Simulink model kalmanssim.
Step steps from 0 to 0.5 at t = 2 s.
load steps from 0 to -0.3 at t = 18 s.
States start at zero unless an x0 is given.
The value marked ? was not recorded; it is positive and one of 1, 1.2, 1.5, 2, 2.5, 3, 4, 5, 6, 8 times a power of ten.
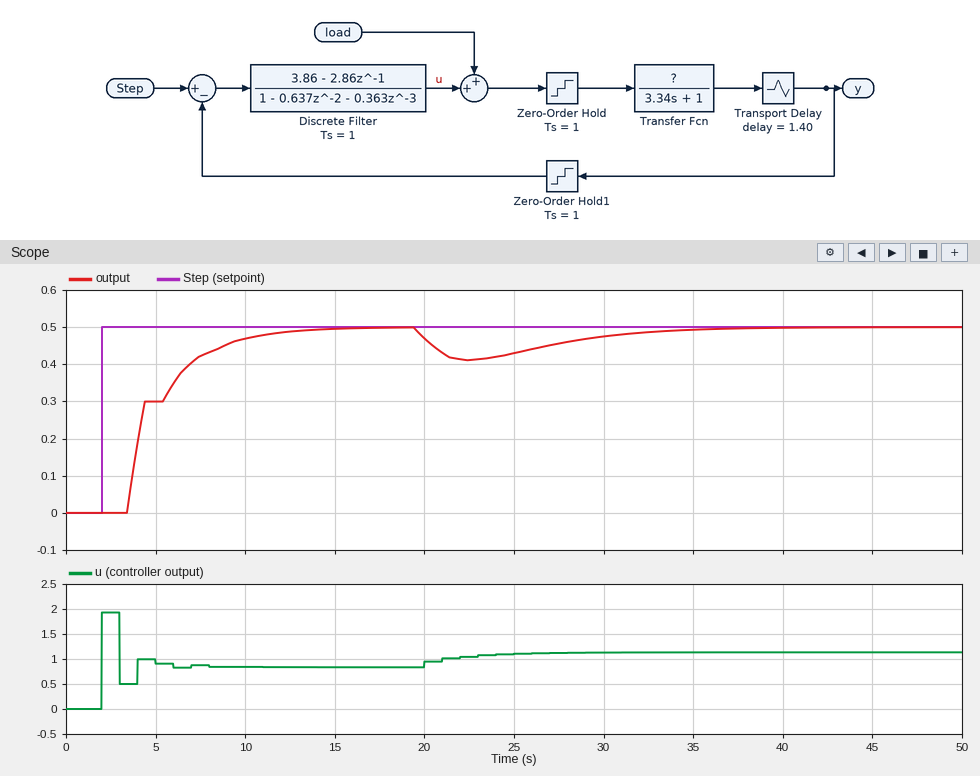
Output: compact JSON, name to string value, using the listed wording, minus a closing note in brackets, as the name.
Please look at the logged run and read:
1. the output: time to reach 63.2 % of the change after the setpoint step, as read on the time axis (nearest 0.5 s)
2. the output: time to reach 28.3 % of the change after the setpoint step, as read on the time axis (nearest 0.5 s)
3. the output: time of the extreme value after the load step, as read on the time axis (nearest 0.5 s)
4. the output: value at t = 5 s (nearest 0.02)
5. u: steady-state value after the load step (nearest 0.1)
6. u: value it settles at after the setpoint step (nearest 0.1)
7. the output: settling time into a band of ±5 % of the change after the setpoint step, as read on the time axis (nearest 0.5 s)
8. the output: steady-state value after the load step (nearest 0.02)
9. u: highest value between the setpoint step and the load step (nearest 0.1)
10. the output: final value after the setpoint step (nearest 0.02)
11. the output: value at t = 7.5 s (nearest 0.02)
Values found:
{"the output: time to reach 63.2 % of the change after the setpoint step, as read on the time axis": "5.5 s", "the output: time to reach 28.3 % of the change after the setpoint step, as read on the time axis": "4.0 s", "the output: time of the extreme value after the load step, as read on the time axis": "22.5 s", "the output: value at t = 5 s": "0.30", "u: steady-state value after the load step": "1.1", "u: value it settles at after the setpoint step": "0.8", "the output: settling time into a band of ±5 % of the change after the setpoint step, as read on the time axis": "10.5 s", "the output: steady-state value after the load step": "0.50", "u: highest value between the setpoint step and the load step": "1.9", "the output: final value after the setpoint step": "0.50", "the output: value at t = 7.5 s": "0.42"}
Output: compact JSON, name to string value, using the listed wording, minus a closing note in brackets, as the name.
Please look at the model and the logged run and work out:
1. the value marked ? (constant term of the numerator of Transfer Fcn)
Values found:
{"the value marked ?": "0.6"}
